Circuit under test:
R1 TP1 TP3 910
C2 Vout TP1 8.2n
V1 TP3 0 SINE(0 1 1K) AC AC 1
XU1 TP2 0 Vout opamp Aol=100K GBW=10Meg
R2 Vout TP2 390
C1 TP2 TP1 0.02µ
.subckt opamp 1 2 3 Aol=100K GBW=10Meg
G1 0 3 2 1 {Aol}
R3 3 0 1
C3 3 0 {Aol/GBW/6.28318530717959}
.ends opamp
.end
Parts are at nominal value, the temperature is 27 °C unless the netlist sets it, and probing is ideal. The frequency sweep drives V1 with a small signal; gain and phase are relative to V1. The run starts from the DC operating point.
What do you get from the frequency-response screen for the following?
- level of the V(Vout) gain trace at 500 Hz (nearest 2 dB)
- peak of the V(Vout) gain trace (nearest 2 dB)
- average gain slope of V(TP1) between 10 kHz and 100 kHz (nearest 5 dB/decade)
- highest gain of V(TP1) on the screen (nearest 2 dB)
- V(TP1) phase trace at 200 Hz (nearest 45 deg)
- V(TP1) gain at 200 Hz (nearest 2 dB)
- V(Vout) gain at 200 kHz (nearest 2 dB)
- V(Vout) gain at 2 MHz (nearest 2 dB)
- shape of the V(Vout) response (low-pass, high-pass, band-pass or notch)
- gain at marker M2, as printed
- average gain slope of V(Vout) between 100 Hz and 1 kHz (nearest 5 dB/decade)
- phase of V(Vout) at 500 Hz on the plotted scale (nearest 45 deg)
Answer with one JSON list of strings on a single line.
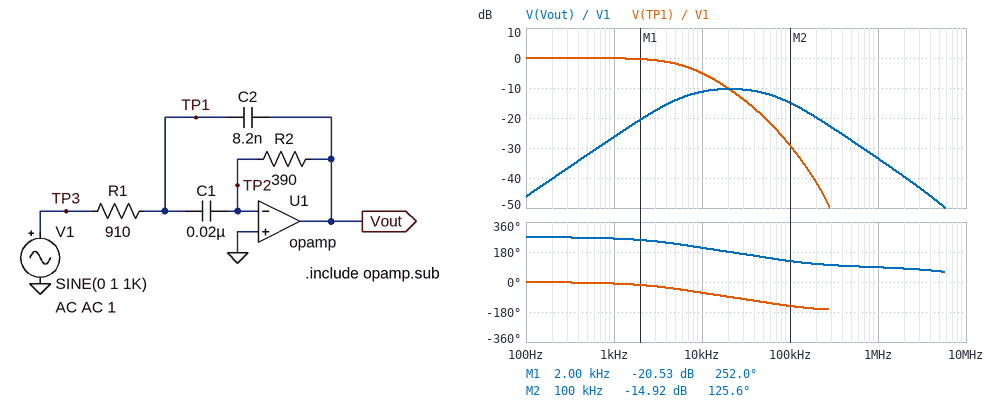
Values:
["-32 dB", "-10 dB", "-25 dB/decade", "0 dB", "0 deg", "0 dB", "-20 dB", "-40 dB", "band-pass", "-14.92 dB", "20 dB/decade", "270 deg"]
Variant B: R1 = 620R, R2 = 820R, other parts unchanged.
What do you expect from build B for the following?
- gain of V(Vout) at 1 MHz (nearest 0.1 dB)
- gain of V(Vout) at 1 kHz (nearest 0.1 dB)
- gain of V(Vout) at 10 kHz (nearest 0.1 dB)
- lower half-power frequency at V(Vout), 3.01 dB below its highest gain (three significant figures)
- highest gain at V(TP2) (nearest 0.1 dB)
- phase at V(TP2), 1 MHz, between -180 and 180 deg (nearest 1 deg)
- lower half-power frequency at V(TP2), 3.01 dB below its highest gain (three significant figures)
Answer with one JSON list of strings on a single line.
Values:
["-30.2 dB", "-19.8 dB", "-1.9 dB", "7.44 kHz", "-50.1 dB", "-4 deg", "25.3 kHz"]
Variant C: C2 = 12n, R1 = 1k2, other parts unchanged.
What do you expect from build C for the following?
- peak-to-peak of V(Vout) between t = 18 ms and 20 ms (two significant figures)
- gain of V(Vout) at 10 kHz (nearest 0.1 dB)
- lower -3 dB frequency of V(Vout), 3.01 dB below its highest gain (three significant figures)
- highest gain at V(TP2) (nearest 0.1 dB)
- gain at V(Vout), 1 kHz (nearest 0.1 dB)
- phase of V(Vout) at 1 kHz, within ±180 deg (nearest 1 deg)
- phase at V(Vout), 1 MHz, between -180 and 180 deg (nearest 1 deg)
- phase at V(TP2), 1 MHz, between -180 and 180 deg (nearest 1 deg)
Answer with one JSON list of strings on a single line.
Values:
["96 mV", "-14.1 dB", "3.87 kHz", "-59.2 dB", "-26.4 dB", "-104 deg", "87 deg", "-3 deg"]
